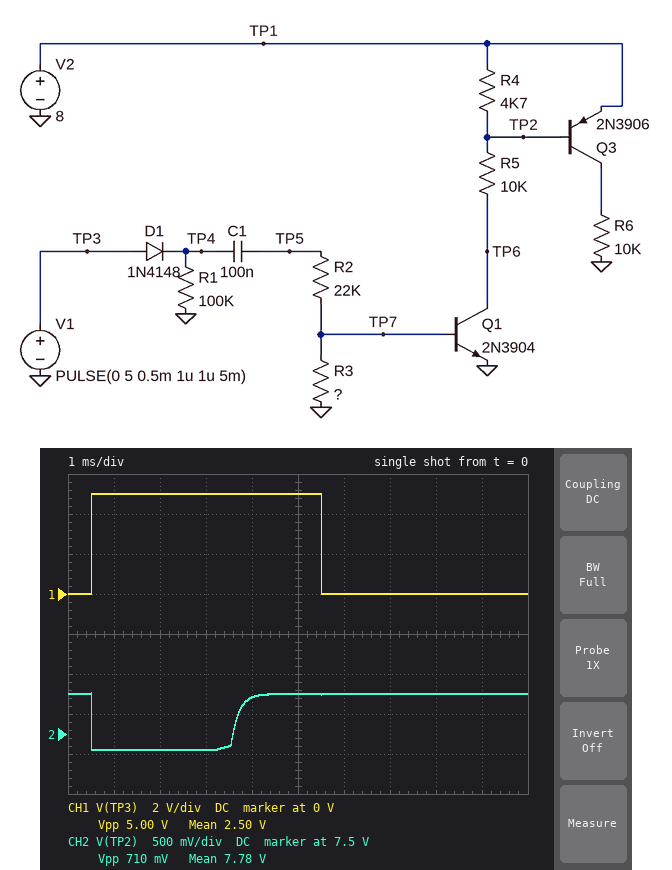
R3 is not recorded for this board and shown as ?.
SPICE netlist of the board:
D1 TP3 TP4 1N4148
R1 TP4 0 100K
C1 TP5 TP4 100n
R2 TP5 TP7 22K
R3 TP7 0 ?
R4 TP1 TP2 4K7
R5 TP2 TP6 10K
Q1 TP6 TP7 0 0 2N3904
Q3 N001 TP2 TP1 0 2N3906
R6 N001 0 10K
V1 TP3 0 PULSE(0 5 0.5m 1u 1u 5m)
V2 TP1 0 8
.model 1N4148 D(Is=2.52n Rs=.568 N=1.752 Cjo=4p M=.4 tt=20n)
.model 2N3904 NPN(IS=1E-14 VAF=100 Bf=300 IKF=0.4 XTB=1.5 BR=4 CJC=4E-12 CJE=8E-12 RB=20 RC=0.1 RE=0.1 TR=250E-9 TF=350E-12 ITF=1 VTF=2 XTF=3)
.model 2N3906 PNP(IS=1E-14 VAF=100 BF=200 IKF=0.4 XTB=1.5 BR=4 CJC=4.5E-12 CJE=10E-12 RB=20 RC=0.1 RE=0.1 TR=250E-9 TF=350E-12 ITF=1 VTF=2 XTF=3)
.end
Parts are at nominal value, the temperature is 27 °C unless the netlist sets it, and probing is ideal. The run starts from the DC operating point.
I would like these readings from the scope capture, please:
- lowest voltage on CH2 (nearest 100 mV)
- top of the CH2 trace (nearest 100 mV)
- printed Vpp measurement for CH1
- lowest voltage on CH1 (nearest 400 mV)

7.3 V
8.0 V
5.00 V
0 V
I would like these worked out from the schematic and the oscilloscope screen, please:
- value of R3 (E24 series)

13 kΩ
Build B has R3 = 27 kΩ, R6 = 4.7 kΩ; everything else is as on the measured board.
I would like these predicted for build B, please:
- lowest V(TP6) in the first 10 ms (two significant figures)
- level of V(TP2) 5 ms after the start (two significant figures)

24 mV
7.3 V
